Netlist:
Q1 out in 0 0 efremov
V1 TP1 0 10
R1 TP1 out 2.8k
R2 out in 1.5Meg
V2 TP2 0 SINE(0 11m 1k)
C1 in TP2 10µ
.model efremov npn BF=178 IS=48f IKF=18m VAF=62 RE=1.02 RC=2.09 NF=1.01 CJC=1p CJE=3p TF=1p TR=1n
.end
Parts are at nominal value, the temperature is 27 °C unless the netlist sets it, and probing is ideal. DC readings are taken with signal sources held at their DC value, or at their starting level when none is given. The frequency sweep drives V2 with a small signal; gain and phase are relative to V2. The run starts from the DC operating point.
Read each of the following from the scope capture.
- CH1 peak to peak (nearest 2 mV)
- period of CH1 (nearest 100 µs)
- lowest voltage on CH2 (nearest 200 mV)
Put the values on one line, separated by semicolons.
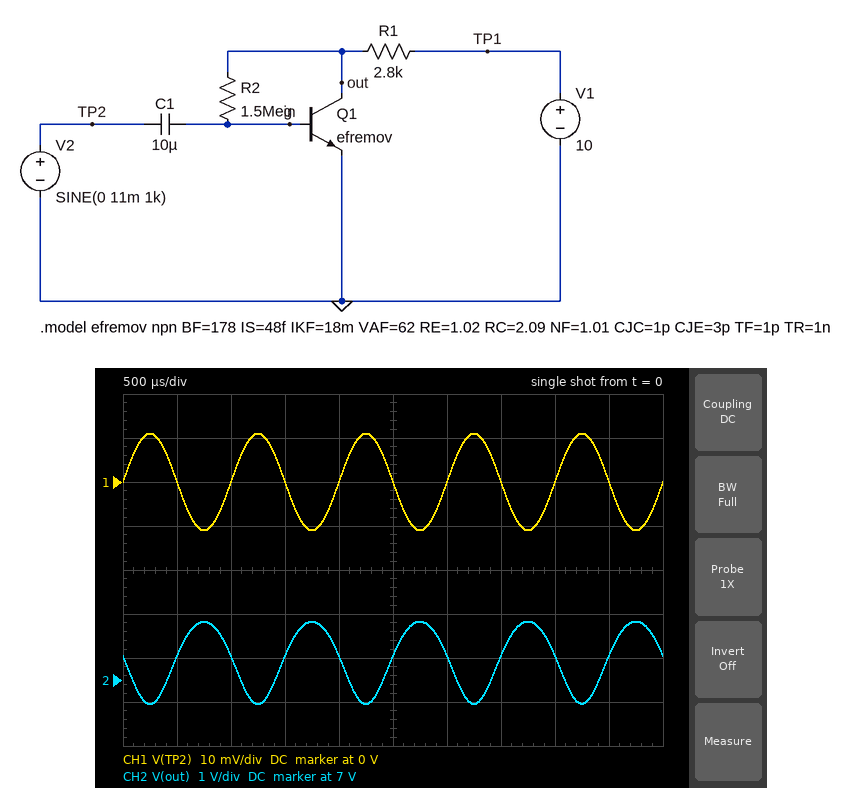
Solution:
22 mV; 1.0 ms; 6.4 V
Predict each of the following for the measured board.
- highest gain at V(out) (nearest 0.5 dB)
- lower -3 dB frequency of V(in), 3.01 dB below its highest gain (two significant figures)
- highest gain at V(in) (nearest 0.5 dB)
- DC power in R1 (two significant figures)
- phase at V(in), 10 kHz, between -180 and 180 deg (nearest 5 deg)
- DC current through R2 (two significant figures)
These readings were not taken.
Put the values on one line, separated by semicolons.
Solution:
38.5 dB; 3.6 Hz; 0 dB; 2.2 mW; 0 deg; 4.6 µA
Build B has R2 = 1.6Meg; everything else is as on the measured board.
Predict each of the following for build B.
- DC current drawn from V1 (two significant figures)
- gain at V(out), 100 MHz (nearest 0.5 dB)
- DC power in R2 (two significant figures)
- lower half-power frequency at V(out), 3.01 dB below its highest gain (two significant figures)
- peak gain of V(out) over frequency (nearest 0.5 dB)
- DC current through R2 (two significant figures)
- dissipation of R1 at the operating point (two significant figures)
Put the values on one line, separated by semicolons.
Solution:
840 µA; 36.0 dB; 31 µW; 3.4 Hz; 38.0 dB; 4.4 µA; 2.0 mW
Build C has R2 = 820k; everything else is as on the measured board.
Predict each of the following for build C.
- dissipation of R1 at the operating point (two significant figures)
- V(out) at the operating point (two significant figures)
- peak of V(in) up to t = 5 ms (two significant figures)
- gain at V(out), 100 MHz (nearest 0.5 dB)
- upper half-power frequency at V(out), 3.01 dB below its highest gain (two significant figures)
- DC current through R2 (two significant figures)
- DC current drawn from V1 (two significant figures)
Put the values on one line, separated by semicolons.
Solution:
4.7 mW; 6.4 V; 640 mV; 39.0 dB; 120 MHz; 7.0 µA; 1.3 mA
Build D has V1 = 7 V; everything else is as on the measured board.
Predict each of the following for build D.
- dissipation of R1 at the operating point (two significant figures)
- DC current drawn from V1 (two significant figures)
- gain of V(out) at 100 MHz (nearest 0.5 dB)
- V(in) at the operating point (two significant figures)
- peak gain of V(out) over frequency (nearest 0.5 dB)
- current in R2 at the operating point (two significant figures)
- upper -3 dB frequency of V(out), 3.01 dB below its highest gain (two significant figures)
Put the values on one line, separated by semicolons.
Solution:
980 µW; 590 µA; 33.0 dB; 610 mV; 35.5 dB; 3.2 µA; 110 MHz
